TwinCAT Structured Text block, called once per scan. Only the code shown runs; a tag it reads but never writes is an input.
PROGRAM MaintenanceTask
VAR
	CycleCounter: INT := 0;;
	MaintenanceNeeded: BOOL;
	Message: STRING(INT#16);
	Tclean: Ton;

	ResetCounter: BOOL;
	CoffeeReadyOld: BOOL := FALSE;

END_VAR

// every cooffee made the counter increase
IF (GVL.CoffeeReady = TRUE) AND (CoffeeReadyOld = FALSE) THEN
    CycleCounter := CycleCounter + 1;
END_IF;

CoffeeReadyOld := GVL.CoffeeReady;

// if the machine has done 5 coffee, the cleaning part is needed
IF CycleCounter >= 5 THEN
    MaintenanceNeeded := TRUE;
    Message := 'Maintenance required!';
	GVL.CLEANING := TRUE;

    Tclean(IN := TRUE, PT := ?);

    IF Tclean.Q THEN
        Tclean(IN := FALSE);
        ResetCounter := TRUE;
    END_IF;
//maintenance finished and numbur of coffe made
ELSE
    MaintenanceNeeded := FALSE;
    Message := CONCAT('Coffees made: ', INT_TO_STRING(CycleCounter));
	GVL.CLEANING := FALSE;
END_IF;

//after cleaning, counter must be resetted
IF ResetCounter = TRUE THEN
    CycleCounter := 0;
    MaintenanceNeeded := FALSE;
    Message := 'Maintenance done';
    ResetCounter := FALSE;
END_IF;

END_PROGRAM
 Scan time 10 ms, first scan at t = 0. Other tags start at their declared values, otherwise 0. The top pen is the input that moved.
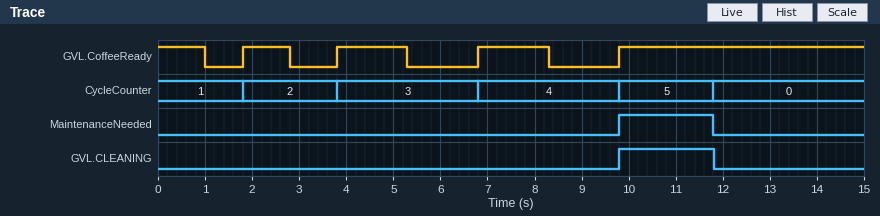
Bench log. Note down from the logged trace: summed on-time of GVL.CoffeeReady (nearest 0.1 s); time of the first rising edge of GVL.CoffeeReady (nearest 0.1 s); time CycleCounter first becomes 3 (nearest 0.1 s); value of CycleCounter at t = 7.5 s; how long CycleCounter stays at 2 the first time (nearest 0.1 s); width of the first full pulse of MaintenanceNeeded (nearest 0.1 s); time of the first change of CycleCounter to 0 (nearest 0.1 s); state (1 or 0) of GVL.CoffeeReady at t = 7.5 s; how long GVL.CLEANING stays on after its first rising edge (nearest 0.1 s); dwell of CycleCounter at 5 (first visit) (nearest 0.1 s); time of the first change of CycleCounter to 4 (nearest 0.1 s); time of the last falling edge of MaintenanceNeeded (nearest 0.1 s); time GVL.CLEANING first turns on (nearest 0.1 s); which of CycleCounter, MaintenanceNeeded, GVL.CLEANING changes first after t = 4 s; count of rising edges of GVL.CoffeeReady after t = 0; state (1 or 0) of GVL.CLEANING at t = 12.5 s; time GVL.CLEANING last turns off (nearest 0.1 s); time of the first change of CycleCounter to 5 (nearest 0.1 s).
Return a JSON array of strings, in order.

["10.2 s", "1.8 s", "3.8 s", "4", "2.0 s", "2.0 s", "11.8 s", "1", "2.0 s", "2.0 s", "6.8 s", "11.8 s", "9.8 s", "CycleCounter", "4", "0", "11.8 s", "9.8 s"]
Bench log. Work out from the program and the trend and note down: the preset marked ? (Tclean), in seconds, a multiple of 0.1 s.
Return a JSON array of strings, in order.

["2.0 s"]
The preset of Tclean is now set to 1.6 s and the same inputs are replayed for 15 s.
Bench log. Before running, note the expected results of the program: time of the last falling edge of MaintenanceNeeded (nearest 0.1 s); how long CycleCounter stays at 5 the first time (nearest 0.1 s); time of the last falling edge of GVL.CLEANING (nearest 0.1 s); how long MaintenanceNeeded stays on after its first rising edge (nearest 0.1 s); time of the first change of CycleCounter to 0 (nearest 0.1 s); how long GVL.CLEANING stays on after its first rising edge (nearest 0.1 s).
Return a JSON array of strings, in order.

["11.4 s", "1.6 s", "11.4 s", "1.6 s", "11.4 s", "1.6 s"]
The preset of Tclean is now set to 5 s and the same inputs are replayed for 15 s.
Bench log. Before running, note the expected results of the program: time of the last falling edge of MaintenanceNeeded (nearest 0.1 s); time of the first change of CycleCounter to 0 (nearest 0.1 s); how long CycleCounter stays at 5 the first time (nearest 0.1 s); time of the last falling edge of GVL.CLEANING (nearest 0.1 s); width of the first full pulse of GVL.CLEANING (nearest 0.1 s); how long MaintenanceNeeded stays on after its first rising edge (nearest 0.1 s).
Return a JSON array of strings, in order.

["14.8 s", "14.8 s", "5.0 s", "14.8 s", "5.0 s", "5.0 s"]
